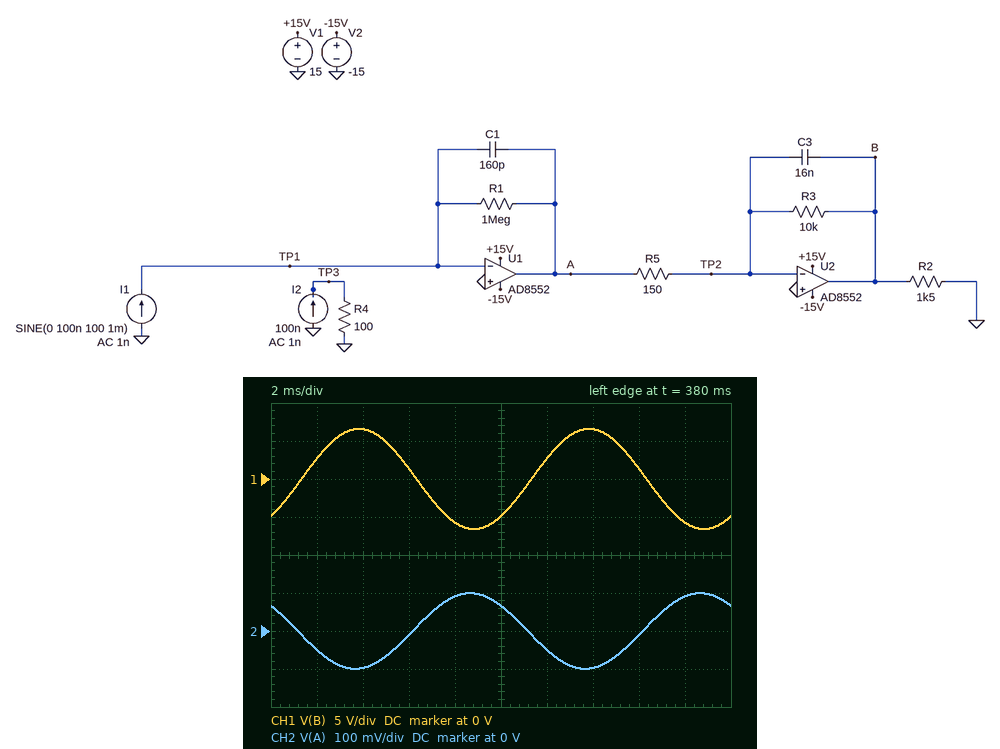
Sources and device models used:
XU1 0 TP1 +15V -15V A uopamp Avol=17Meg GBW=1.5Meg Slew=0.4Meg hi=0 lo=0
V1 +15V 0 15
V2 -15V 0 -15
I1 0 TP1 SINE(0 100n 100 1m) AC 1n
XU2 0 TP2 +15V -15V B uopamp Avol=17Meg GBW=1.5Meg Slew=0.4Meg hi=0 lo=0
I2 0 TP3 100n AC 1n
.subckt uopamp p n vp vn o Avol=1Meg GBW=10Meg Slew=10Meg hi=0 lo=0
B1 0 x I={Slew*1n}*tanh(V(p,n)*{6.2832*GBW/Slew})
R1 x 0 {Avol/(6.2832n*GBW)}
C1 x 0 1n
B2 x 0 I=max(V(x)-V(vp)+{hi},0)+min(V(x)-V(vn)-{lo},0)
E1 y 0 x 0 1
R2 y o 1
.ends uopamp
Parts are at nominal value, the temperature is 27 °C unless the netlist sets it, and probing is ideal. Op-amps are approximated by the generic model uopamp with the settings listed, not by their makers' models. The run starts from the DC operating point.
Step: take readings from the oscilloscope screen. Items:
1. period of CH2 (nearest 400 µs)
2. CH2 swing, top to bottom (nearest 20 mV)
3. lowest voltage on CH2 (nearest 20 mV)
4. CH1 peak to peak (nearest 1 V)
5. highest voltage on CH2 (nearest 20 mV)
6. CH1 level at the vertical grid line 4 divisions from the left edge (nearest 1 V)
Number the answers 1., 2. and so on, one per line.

1. 10.0 ms
2. 200 mV
3. -100 mV
4. 13 V
5. 100 mV
6. -6 V
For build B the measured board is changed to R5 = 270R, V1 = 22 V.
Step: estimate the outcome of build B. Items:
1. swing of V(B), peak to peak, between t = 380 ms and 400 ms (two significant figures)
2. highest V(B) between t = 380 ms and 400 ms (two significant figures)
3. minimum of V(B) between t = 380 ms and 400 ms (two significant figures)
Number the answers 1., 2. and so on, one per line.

1. 7.3 V
2. 3.7 V
3. -3.7 V
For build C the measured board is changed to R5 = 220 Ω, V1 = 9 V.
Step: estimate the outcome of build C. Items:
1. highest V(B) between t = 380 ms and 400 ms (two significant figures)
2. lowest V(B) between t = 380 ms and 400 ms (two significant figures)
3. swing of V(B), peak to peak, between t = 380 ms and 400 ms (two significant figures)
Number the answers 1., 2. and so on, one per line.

1. 4.5 V
2. -4.5 V
3. 9.0 V
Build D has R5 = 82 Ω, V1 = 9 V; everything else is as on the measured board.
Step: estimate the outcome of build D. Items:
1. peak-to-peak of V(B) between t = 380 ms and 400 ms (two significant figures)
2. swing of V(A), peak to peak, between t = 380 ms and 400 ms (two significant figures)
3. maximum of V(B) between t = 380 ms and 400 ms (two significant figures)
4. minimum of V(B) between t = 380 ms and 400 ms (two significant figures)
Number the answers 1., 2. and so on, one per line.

1. 21 V
2. 200 mV
3. 9.0 V
4. -12 V
